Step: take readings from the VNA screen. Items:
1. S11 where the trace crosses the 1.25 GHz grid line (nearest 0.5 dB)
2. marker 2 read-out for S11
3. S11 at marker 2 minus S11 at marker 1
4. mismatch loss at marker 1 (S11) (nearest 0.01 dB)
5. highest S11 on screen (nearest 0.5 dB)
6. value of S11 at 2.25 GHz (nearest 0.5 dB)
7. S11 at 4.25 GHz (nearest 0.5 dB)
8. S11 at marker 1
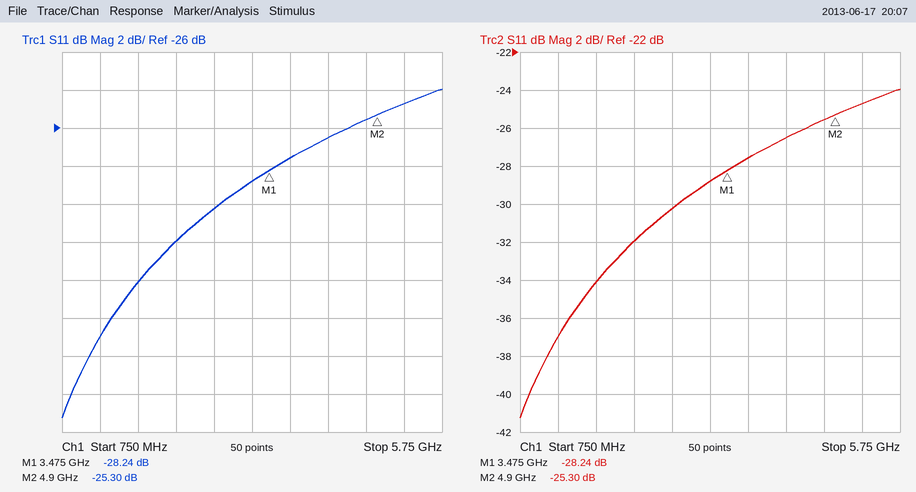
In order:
-37.0 dB
-25.30 dB
2.94 dB
0.01 dB
-24.0 dB
-32.0 dB
-26.5 dB
-28.24 dB
